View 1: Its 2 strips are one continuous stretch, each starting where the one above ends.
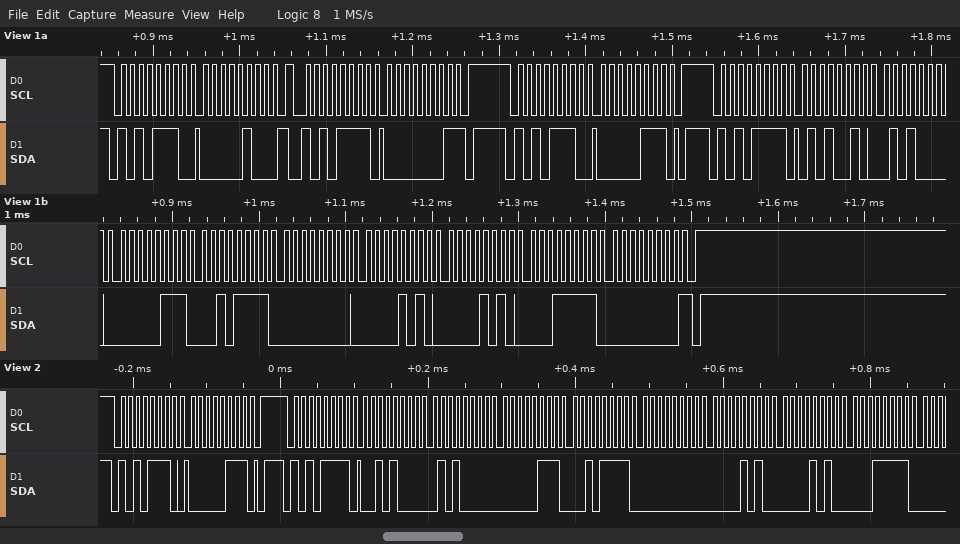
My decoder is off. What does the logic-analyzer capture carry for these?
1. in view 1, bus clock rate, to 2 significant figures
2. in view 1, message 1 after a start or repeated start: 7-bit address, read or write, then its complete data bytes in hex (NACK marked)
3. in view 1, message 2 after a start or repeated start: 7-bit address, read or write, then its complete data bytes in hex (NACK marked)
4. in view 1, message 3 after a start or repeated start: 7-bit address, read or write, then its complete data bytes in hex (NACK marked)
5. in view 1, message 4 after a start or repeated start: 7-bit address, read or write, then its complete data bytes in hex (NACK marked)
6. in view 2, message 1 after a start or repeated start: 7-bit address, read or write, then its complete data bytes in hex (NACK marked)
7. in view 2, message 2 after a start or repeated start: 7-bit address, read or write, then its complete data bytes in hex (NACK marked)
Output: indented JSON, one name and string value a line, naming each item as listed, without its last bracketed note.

{
  "in view 1, bus clock rate, to 2 significant figures": "100 kHz",
  "in view 1, message 1 after a start or repeated start: 7-bit address, read or write, then its complete data bytes in hex": "0x57 write: 04",
  "in view 1, message 2 after a start or repeated start: 7-bit address, read or write, then its complete data bytes in hex": "0x57 read: 01 NACK",
  "in view 1, message 3 after a start or repeated start: 7-bit address, read or write, then its complete data bytes in hex": "0x57 write: 07",
  "in view 1, message 4 after a start or repeated start: 7-bit address, read or write, then its complete data bytes in hex": "0x57 read: 52 50 07 2F 00 0A 0A 1F 00 NACK",
  "in view 2, message 1 after a start or repeated start: 7-bit address, read or write, then its complete data bytes in hex": "0x57 write: 07",
  "in view 2, message 2 after a start or repeated start: 7-bit address, read or write, then its complete data bytes in hex": "0x57 read: 28 50 07 2F 00 0A 0A 1F"
}
